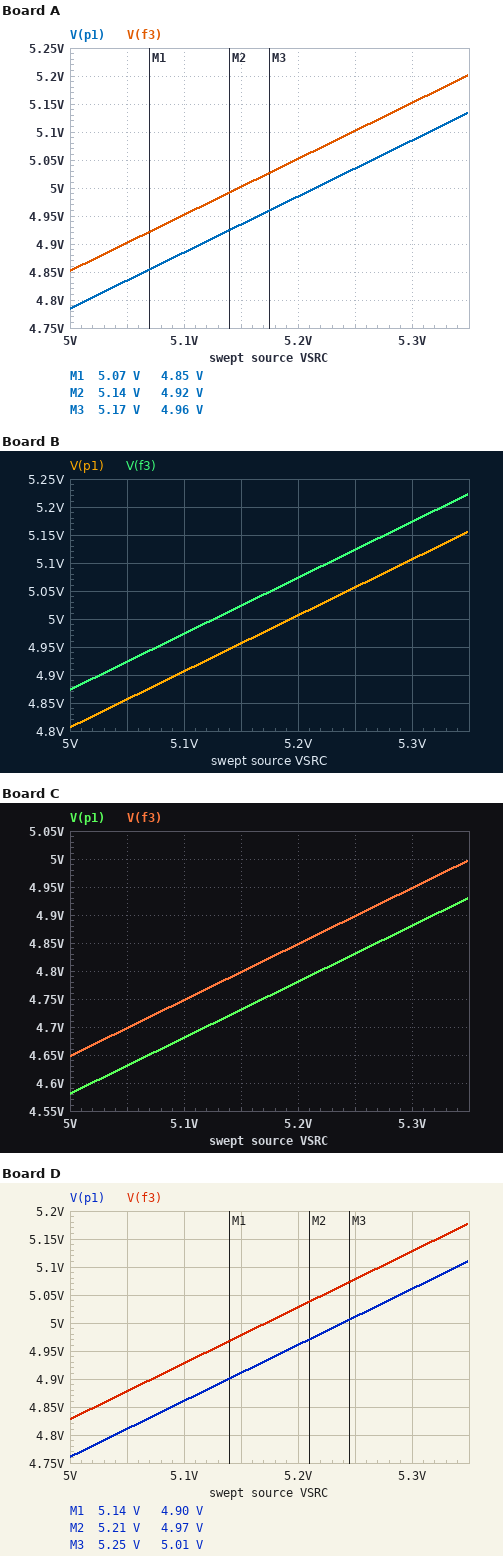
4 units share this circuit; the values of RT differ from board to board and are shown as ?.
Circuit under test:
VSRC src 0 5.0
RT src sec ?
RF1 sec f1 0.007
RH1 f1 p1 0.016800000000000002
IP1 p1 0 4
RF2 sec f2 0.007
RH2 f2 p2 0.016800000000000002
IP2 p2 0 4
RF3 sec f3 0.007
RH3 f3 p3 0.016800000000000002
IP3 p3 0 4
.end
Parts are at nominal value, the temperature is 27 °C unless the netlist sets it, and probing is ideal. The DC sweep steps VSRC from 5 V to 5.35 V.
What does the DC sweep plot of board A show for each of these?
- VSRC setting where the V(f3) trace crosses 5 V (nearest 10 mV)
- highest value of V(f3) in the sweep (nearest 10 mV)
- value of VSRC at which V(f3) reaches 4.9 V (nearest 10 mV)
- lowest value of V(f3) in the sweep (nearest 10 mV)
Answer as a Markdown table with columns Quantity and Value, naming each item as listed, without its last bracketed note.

| Quantity | Value |
|---|---|
| VSRC setting where the V(f3) trace crosses 5 V | 5.15 V |
| highest value of V(f3) in the sweep | 5.20 V |
| value of VSRC at which V(f3) reaches 4.9 V | 5.05 V |
| lowest value of V(f3) in the sweep | 4.85 V |
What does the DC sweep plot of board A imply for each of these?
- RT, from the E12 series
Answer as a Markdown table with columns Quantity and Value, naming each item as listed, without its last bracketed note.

| Quantity | Value |
|---|---|
| RT, from the E12 series | 0.01 Ω |
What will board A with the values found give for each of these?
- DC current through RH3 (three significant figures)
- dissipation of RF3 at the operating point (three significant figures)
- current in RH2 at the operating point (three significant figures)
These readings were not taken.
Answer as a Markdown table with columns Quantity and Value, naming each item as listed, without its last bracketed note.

| Quantity | Value |
|---|---|
| DC current through RH3 | 4.00 A |
| dissipation of RF3 at the operating point | 112 mW |
| current in RH2 at the operating point | 4.00 A |
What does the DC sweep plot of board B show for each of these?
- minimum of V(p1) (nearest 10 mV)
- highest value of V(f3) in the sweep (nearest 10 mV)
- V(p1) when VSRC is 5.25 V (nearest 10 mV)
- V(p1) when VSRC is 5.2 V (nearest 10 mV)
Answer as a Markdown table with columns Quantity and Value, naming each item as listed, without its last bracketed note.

| Quantity | Value |
|---|---|
| minimum of V(p1) | 4.81 V |
| highest value of V(f3) in the sweep | 5.22 V |
| V(p1) when VSRC is 5.25 V | 5.06 V |
| V(p1) when VSRC is 5.2 V | 5.01 V |
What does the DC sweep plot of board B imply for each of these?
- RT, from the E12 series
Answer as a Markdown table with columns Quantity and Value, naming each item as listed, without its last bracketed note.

| Quantity | Value |
|---|---|
| RT, from the E12 series | 8.2 mΩ |
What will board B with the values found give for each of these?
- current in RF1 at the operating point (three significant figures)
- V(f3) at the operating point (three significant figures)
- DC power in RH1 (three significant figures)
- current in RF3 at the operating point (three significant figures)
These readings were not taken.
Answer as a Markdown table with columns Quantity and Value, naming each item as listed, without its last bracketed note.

| Quantity | Value |
|---|---|
| current in RF1 at the operating point | 4.00 A |
| V(f3) at the operating point | 4.87 V |
| DC power in RH1 | 269 mW |
| current in RF3 at the operating point | 4.00 A |
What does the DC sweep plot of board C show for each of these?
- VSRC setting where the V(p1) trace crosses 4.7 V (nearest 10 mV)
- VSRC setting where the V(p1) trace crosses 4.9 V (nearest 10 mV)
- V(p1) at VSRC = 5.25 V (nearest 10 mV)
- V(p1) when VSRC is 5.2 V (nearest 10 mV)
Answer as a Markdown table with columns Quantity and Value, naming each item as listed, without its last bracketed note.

| Quantity | Value |
|---|---|
| VSRC setting where the V(p1) trace crosses 4.7 V | 5.12 V |
| VSRC setting where the V(p1) trace crosses 4.9 V | 5.32 V |
| V(p1) at VSRC = 5.25 V | 4.83 V |
| V(p1) when VSRC is 5.2 V | 4.78 V |
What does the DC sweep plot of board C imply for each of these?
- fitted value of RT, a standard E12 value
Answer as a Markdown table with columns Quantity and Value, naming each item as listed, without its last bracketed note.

| Quantity | Value |
|---|---|
| fitted value of RT, a standard E12 value | 0.027 Ω |
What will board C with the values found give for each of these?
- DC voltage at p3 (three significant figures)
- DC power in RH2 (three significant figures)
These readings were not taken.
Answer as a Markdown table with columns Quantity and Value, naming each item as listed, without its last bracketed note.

| Quantity | Value |
|---|---|
| DC voltage at p3 | 4.58 V |
| DC power in RH2 | 269 mW |
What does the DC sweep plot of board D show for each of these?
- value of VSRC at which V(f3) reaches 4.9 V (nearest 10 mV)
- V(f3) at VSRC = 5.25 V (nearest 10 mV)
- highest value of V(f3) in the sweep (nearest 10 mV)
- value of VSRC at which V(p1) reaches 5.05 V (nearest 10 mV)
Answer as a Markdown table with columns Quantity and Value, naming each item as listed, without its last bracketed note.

| Quantity | Value |
|---|---|
| value of VSRC at which V(f3) reaches 4.9 V | 5.07 V |
| V(f3) at VSRC = 5.25 V | 5.08 V |
| highest value of V(f3) in the sweep | 5.18 V |
| value of VSRC at which V(p1) reaches 5.05 V | 5.29 V |
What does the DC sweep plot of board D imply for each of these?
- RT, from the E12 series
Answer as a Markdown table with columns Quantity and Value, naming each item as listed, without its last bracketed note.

| Quantity | Value |
|---|---|
| RT, from the E12 series | 0.012 Ω |
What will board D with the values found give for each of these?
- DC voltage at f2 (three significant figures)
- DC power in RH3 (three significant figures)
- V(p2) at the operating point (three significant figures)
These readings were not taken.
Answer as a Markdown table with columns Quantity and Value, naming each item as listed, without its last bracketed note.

| Quantity | Value |
|---|---|
| DC voltage at f2 | 4.83 V |
| DC power in RH3 | 269 mW |
| V(p2) at the operating point | 4.76 V |
